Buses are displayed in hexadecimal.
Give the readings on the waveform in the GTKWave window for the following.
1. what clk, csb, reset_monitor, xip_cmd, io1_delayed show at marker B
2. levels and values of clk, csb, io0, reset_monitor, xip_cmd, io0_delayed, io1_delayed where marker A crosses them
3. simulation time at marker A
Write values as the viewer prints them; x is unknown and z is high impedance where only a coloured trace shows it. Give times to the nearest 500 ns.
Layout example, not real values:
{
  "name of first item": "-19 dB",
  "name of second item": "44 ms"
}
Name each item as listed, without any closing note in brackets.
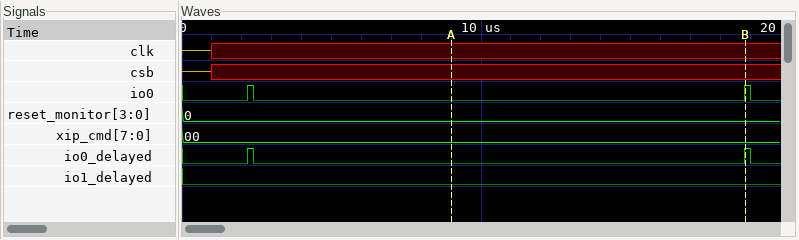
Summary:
{
  "what clk, csb, reset_monitor, xip_cmd, io1_delayed show at marker B": "clk=x, csb=x, reset_monitor=0, xip_cmd=00, io1_delayed=0",
  "levels and values of clk, csb, io0, reset_monitor, xip_cmd, io0_delayed, io1_delayed where marker A crosses them": "clk=x, csb=x, io0=0, reset_monitor=0, xip_cmd=00, io0_delayed=0, io1_delayed=0",
  "simulation time at marker A": "9000 ns"
}
